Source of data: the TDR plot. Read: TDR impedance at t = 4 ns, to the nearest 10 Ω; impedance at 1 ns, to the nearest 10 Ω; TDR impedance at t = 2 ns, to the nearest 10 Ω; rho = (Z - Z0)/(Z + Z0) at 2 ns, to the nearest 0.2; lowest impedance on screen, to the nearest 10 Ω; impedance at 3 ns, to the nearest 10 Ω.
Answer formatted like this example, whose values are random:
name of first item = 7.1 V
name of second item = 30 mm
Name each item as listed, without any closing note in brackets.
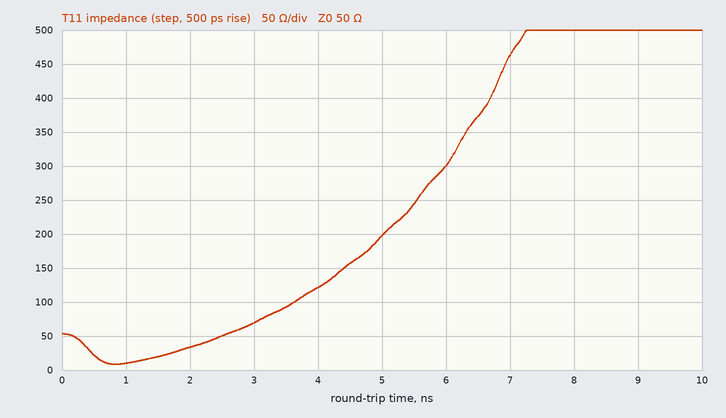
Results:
TDR impedance at t = 4 ns, to the nearest 10 Ω = 120 Ω
impedance at 1 ns, to the nearest 10 Ω = 10 Ω
TDR impedance at t = 2 ns, to the nearest 10 Ω = 30 Ω
rho = (Z - Z0)/(Z + Z0) at 2 ns, to the nearest 0.2 = -0.2
lowest impedance on screen, to the nearest 10 Ω = 10 Ω
impedance at 3 ns, to the nearest 10 Ω = 70 Ω
